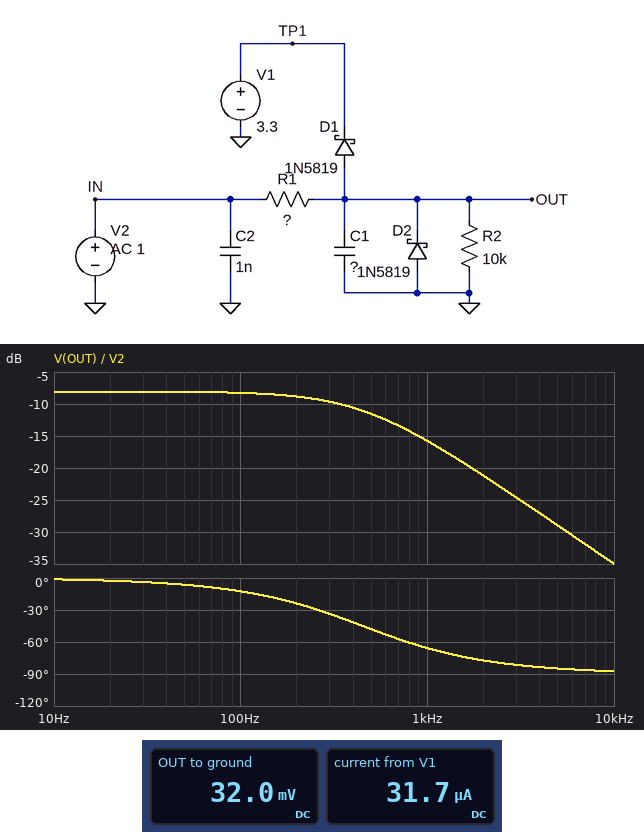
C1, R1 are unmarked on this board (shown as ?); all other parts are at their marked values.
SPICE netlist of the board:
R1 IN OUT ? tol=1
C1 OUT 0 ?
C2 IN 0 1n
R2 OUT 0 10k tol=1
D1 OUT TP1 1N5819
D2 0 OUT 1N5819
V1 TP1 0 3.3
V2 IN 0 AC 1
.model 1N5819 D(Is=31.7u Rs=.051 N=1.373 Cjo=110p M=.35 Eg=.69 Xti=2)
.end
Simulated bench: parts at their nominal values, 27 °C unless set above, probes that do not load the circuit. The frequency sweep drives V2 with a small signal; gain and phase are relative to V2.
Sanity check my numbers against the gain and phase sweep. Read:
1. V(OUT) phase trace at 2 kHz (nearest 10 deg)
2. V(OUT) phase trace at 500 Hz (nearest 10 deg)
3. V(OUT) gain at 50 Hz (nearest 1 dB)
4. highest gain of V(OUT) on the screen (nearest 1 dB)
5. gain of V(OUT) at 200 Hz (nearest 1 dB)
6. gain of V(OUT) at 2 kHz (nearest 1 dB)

-80 deg
-50 deg
-8 dB
-8 dB
-9 dB
-21 dB
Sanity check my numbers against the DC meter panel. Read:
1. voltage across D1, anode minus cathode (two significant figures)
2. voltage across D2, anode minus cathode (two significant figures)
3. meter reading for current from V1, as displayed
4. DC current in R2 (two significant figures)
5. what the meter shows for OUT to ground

-3.3 V
-32 mV
31.7 µA
3.2 µA
32.0 mV
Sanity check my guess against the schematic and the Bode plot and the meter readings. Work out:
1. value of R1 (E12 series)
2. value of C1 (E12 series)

3.3 kΩ
270 nF
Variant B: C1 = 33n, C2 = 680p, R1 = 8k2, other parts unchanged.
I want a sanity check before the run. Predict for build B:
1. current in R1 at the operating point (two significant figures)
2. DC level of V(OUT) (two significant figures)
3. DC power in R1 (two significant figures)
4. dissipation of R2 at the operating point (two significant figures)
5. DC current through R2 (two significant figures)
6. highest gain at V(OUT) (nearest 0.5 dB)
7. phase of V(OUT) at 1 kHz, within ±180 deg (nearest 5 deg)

5.2 µA
43 mV
220 nW
180 nW
4.3 µA
-12.0 dB
-25 deg
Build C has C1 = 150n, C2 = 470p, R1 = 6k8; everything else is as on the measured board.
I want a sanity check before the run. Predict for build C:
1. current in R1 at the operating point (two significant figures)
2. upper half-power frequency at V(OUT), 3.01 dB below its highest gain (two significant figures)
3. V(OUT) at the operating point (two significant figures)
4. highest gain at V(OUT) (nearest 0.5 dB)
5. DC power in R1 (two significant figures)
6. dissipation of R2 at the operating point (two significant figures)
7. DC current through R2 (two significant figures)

6.0 µA
560 Hz
41 mV
-11.0 dB
240 nW
170 nW
4.1 µA
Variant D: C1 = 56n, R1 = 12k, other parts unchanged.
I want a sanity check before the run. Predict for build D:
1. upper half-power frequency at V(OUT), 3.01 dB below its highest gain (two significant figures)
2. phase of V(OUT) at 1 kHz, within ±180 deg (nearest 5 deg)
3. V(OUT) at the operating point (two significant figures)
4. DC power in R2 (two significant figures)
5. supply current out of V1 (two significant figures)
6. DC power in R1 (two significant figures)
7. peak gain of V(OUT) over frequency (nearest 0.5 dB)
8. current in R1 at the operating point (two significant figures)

1.2 kHz
-40 deg
47 mV
220 nW
32 µA
180 nW
-14.0 dB
3.9 µA
